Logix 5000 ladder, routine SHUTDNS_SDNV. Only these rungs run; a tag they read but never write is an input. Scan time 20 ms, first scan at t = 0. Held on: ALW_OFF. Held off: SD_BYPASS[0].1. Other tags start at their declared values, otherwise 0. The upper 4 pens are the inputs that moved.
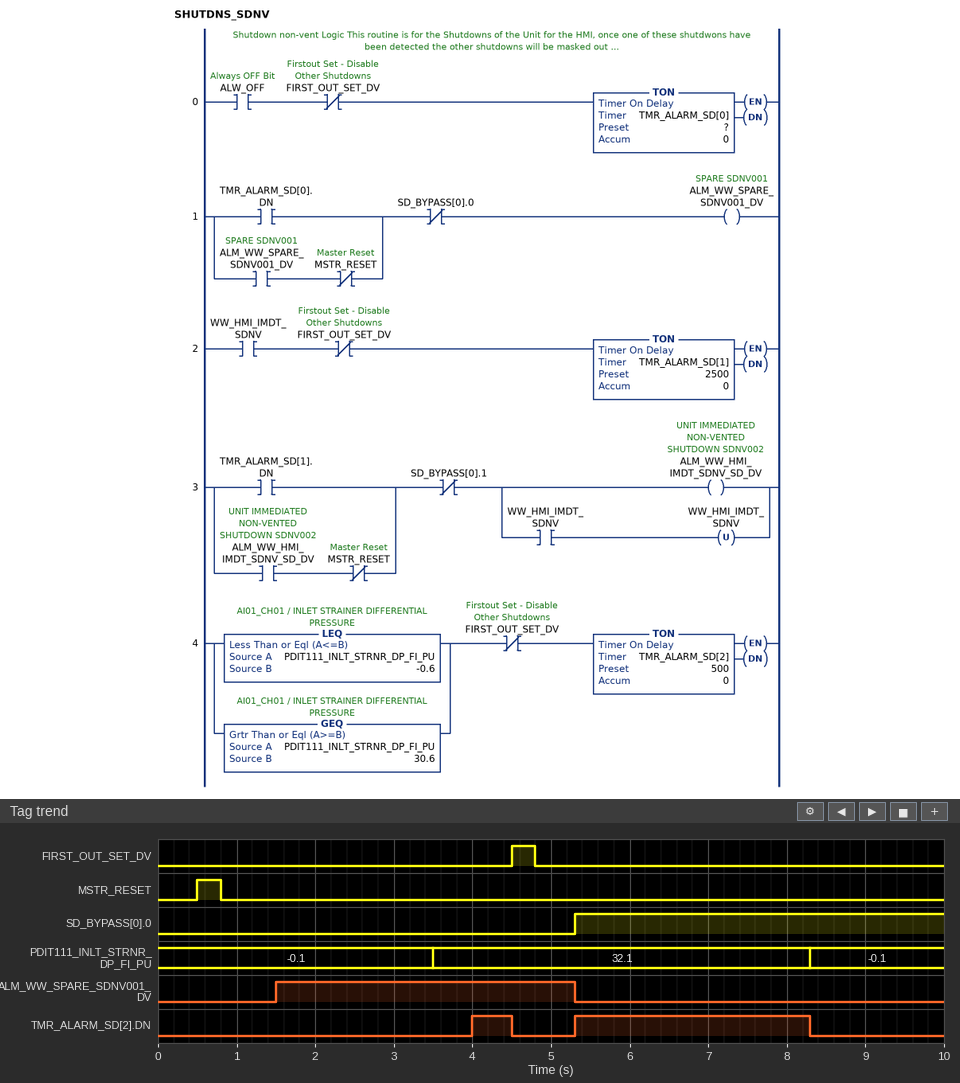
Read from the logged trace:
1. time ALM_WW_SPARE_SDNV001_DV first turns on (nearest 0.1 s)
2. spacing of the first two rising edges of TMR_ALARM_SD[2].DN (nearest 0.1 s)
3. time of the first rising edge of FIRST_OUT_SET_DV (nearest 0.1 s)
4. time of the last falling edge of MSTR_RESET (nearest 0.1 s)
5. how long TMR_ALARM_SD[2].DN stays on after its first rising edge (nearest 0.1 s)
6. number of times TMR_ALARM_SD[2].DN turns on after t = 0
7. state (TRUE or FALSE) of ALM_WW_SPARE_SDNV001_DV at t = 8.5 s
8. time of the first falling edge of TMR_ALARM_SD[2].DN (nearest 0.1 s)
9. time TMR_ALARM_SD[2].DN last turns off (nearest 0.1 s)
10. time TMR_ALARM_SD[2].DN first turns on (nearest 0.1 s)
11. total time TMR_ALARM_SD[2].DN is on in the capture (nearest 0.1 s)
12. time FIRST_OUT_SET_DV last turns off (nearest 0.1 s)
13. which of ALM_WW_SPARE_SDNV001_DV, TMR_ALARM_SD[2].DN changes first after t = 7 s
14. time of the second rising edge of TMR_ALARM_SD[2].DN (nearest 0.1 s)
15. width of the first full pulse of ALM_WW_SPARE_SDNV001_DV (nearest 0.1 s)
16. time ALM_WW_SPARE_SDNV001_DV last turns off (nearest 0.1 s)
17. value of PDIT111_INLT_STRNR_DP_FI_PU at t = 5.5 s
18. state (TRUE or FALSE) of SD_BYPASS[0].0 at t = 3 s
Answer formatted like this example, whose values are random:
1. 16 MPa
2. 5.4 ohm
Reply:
1. 1.5 s
2. 1.3 s
3. 4.5 s
4. 0.8 s
5. 0.5 s
6. 2
7. FALSE
8. 4.5 s
9. 8.3 s
10. 4.0 s
11. 3.5 s
12. 4.8 s
13. TMR_ALARM_SD[2].DN
14. 5.3 s
15. 3.8 s
16. 5.3 s
17. 32.1
18. FALSE
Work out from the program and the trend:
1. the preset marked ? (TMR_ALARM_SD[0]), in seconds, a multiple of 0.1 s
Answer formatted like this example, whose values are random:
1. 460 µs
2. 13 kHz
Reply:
1. 1.5 s
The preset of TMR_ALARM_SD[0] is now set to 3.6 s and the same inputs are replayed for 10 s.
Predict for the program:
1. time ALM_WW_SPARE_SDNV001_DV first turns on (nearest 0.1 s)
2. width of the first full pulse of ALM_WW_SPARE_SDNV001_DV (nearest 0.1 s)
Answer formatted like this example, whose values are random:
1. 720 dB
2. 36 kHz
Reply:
1. 3.6 s
2. 1.7 s
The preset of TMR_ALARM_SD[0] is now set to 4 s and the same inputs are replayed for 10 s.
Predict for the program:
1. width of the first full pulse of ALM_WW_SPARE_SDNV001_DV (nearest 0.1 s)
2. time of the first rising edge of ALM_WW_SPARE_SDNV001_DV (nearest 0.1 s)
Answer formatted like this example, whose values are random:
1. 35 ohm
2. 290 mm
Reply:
1. 1.3 s
2. 4.0 s
